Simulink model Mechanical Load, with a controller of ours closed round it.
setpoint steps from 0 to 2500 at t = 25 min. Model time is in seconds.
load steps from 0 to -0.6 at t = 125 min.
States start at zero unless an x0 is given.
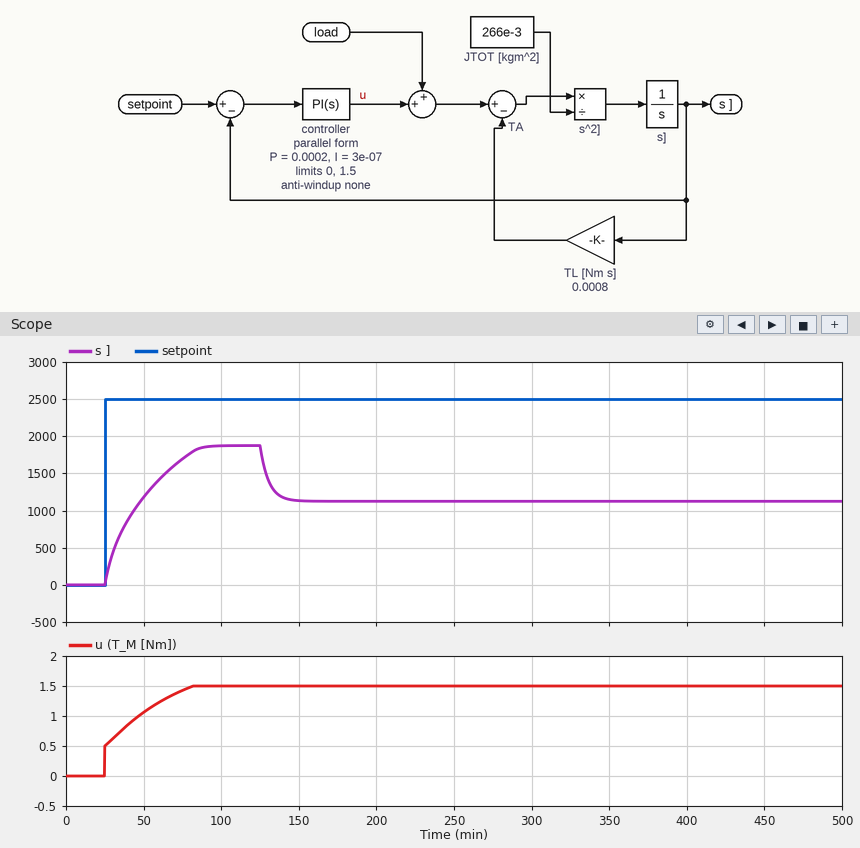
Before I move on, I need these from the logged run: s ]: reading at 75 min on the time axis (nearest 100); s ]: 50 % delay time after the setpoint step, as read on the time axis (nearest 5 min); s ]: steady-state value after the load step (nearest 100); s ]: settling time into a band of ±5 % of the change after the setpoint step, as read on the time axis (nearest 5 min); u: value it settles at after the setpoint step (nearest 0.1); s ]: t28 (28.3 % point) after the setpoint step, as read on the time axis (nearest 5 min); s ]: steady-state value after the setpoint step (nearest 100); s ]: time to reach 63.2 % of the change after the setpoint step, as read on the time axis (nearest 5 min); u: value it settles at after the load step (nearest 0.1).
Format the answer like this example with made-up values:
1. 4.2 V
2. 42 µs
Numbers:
1. 1700
2. 40 min
3. 1100
4. 80 min
5. 1.5
6. 30 min
7. 1900
8. 50 min
9. 1.5
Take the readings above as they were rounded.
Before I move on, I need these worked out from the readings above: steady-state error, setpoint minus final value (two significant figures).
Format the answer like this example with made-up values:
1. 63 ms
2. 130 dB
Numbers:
1. 600
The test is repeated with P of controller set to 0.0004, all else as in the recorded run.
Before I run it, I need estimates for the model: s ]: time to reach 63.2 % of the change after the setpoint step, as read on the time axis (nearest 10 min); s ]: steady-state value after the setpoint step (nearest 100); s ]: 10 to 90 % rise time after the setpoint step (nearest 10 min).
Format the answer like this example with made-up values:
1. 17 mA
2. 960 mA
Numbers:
1. 40 min
2. 1900
3. 50 min
